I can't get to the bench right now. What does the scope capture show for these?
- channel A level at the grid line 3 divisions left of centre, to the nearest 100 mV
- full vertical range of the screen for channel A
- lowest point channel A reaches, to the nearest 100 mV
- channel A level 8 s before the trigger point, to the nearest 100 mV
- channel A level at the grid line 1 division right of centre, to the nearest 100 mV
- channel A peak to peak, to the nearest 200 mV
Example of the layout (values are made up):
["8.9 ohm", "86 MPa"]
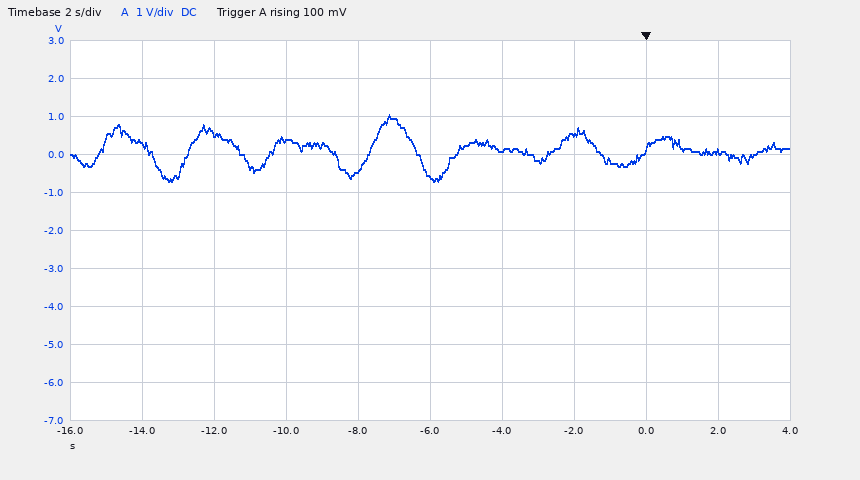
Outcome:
["600 mV", "10 V", "-700 mV", "-400 mV", "100 mV", "1.8 V"]
